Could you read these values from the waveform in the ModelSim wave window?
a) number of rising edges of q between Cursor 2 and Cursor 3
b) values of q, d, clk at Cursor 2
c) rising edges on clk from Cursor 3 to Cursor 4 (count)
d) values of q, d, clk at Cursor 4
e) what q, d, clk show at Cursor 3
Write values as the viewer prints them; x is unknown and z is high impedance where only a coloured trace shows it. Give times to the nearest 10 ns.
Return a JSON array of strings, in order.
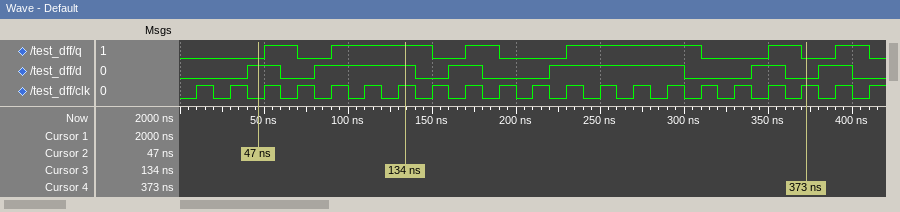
["2", "q=0, d=1, clk=0", "12", "q=0, d=0, clk=1", "q=1, d=1, clk=1"]
